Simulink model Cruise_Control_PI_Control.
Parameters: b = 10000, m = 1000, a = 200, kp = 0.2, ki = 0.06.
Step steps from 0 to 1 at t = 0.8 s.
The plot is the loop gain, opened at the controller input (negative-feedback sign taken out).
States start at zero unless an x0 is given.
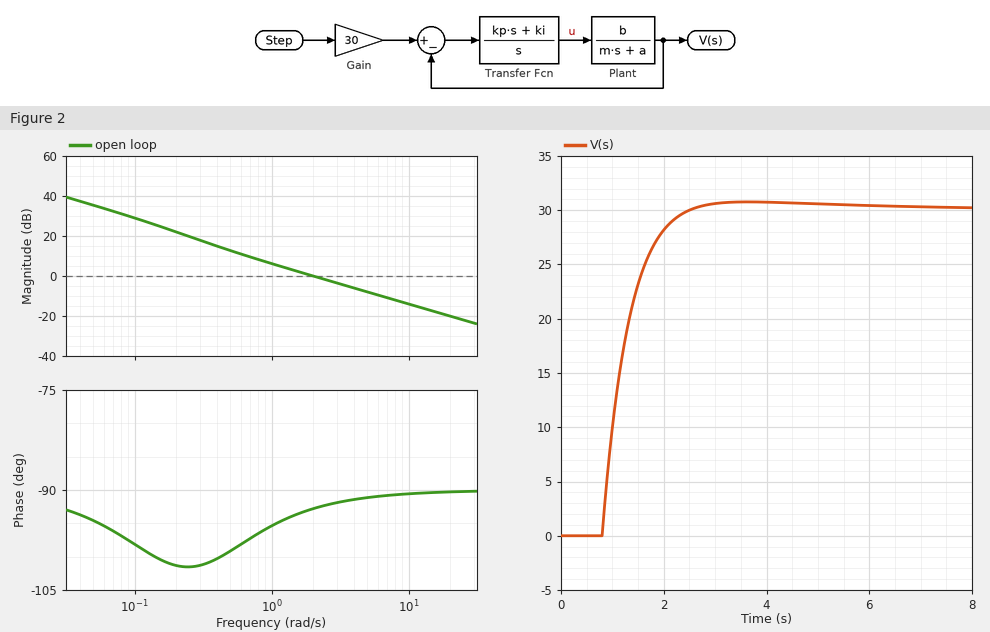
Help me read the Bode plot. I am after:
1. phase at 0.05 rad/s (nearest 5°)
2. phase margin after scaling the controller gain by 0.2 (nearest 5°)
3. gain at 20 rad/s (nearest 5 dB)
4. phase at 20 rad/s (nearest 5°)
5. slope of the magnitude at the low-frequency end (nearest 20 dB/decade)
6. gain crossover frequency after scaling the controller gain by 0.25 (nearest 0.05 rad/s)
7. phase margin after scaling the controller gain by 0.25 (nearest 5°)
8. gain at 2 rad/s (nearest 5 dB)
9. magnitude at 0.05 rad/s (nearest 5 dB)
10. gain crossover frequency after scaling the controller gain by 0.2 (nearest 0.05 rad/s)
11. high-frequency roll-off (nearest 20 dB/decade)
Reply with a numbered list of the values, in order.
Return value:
1. -95°
2. 80°
3. -20 dB
4. -90°
5. -20 dB/decade
6. 0.55 rad/s
7. 80°
8. 0 dB
9. 35 dB
10. 0.45 rad/s
11. -20 dB/decade
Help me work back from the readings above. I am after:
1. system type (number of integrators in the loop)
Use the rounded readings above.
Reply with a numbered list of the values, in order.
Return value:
1. 1
